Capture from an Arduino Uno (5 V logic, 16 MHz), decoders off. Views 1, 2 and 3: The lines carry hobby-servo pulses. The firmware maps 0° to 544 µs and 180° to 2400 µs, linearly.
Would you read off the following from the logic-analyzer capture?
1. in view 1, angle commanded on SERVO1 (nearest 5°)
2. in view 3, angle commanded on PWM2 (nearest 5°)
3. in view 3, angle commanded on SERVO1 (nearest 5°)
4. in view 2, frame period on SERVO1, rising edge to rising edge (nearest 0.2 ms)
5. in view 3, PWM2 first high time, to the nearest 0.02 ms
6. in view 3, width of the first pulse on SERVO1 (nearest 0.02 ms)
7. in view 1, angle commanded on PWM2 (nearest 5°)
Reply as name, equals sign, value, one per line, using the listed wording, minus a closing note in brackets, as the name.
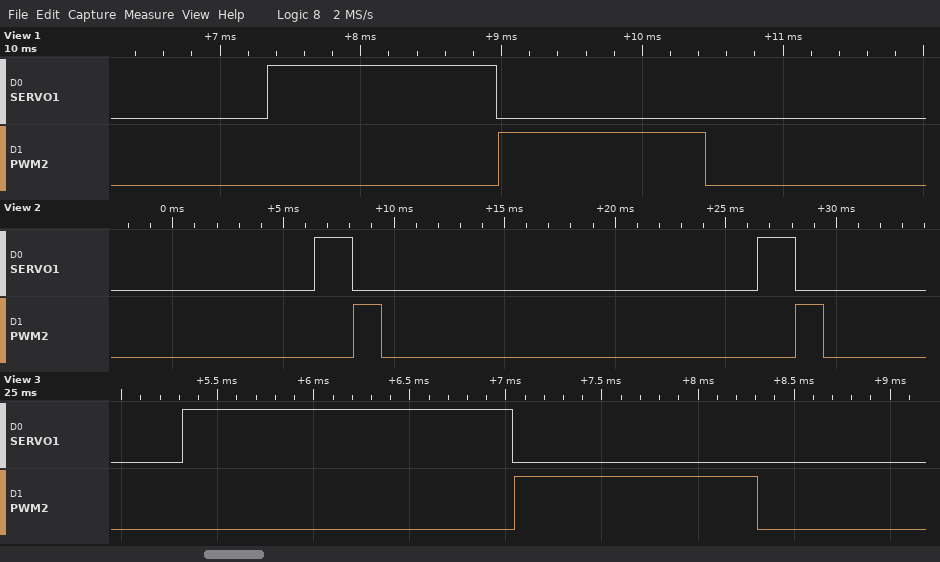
in view 1, angle commanded on SERVO1 = 105°
in view 3, angle commanded on PWM2 = 70°
in view 3, angle commanded on SERVO1 = 115°
in view 2, frame period on SERVO1, rising edge to rising edge = 20.0 ms
in view 3, PWM2 first high time, to the nearest 0.02 ms = 1.26 ms
in view 3, width of the first pulse on SERVO1 = 1.72 ms
in view 1, angle commanded on PWM2 = 90°
